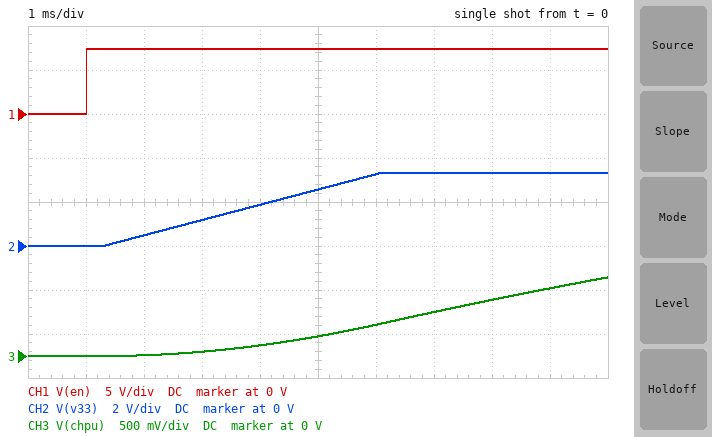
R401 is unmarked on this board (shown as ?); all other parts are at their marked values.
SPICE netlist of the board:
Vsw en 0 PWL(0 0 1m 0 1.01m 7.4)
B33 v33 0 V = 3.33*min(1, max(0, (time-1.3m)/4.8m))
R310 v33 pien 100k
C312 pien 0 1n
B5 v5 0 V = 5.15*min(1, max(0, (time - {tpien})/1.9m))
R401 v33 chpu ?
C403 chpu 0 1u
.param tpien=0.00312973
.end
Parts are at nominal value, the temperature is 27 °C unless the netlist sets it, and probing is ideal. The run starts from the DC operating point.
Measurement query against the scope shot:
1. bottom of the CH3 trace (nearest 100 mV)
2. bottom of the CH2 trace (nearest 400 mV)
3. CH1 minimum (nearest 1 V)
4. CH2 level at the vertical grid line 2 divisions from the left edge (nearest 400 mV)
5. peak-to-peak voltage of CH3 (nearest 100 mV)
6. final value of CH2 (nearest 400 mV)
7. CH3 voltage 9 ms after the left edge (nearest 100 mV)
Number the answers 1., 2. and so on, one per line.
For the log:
1. 0 V
2. 0 V
3. 0 V
4. 400 mV
5. 900 mV
6. 3.2 V
7. 800 mV
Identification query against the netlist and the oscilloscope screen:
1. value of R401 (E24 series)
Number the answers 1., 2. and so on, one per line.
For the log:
1. 20 kΩ
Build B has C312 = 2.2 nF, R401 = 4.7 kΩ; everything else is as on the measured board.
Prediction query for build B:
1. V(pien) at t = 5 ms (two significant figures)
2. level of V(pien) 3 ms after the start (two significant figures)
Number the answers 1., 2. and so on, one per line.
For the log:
1. 2.4 V
2. 1.0 V
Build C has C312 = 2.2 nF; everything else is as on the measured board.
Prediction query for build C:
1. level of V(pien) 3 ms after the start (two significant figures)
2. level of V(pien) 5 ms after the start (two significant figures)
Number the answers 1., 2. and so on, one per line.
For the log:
1. 1.0 V
2. 2.4 V
